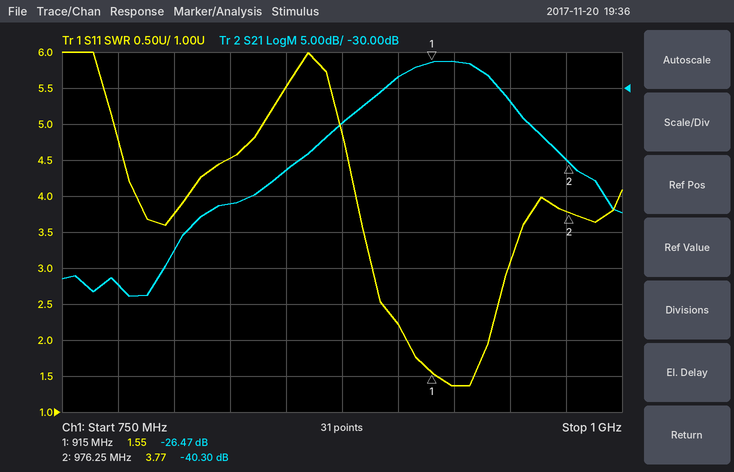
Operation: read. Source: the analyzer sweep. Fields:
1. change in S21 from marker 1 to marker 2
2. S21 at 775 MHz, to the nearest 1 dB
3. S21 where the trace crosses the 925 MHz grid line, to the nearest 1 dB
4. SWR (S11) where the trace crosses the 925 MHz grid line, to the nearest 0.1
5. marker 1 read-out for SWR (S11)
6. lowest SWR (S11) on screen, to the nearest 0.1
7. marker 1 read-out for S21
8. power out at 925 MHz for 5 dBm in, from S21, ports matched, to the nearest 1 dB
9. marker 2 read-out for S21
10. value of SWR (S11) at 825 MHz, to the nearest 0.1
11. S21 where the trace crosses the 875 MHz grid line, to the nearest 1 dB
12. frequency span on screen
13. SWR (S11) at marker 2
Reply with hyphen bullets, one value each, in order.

- -13.83 dB
- -57 dB
- -26 dB
- 1.4
- 1.55
- 1.4
- -26.47 dB
- -21 dBm
- -40.30 dB
- 4.5
- -35 dB
- 250 MHz
- 3.77
